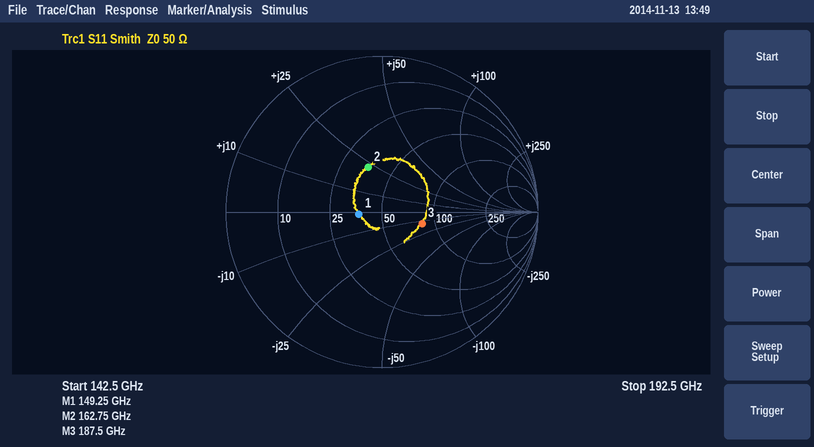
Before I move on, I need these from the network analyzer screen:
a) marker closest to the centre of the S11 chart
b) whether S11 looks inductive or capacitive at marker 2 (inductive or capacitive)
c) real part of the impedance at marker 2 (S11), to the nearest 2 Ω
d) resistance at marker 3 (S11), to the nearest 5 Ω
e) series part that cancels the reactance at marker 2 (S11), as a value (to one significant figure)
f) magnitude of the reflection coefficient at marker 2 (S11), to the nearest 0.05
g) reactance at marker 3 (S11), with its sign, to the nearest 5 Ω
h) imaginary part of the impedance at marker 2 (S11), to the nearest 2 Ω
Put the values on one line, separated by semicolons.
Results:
marker 1; inductive; 36 Ω; 85 Ω; 40 fF; 0.30; -15 Ω; +22 Ω
